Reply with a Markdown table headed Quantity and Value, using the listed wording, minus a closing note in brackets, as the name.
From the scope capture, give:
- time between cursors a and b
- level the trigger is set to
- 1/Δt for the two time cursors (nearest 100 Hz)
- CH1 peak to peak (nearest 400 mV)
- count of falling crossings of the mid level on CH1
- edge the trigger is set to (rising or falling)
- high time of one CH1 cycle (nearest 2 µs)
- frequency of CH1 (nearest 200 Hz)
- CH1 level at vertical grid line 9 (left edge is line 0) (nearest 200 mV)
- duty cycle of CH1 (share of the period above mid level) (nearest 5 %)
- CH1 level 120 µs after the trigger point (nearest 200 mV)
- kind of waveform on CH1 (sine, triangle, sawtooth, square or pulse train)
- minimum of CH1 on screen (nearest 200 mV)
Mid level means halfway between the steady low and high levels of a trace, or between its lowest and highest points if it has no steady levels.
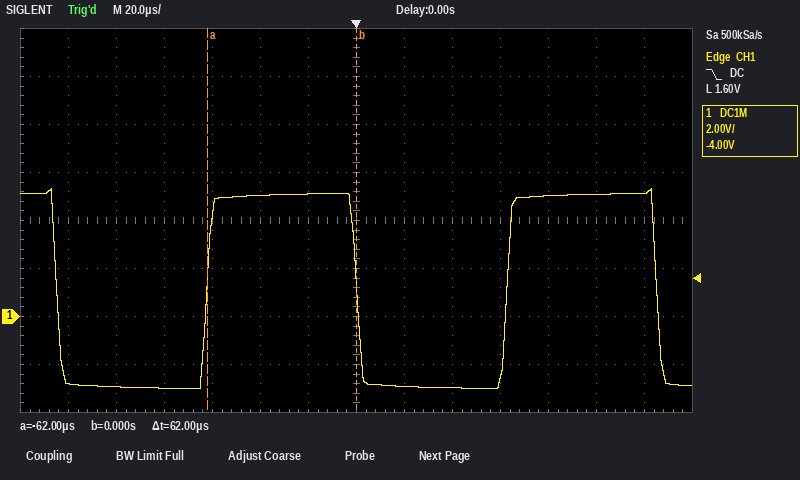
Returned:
| Quantity | Value |
|---|---|
| time between cursors a and b | 62 µs |
| level the trigger is set to | 1.60 V |
| 1/Δt for the two time cursors | 16.1 kHz |
| CH1 peak to peak | 8.4 V |
| count of falling crossings of the mid level on CH1 | 3 |
| edge the trigger is set to | falling |
| high time of one CH1 cycle | 62 µs |
| frequency of CH1 | 8.0 kHz |
| CH1 level at vertical grid line 9 (left edge is line 0) | -3.0 V |
| duty cycle of CH1 (share of the period above mid level) | 50 % |
| CH1 level 120 µs after the trigger point | 5.2 V |
| kind of waveform on CH1 | square |
| minimum of CH1 on screen | -3.0 V |
